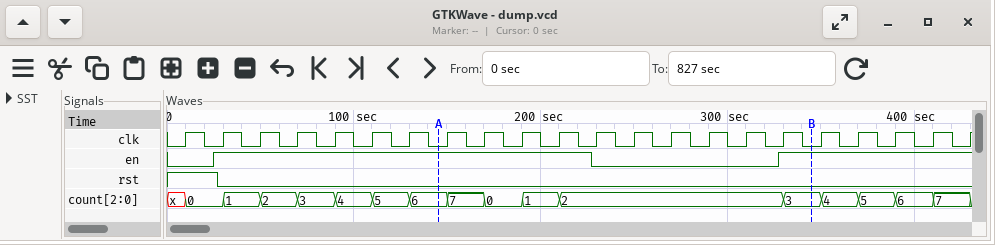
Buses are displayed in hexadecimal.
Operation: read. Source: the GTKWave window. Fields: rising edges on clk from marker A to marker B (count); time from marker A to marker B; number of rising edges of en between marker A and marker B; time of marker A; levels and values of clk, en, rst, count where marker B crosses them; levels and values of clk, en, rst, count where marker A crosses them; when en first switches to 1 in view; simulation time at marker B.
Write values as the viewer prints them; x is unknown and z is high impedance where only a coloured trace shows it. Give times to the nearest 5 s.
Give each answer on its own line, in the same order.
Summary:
10
200 s
1
145 s
clk=0, en=1, rst=0, count=3
clk=0, en=1, rst=0, count=6
25 s
345 s
